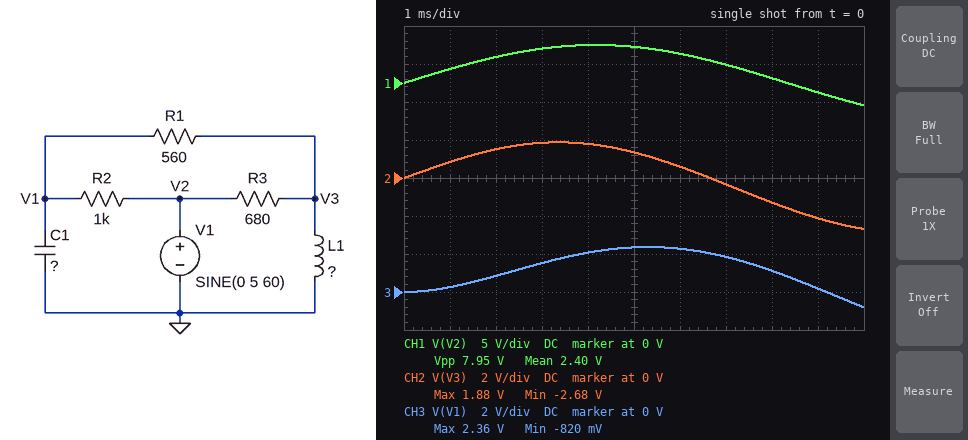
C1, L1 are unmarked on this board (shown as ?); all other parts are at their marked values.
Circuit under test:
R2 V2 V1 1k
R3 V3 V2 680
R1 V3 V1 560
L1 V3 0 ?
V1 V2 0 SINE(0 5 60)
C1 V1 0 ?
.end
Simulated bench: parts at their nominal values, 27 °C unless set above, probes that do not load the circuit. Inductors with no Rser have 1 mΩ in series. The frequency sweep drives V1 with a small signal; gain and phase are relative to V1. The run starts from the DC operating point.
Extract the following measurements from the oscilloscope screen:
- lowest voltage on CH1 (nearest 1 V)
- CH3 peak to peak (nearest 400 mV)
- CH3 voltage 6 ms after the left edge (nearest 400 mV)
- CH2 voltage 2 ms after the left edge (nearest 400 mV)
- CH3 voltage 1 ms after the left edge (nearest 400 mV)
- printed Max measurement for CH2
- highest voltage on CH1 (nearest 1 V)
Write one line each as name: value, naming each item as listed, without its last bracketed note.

lowest voltage on CH1: -3 V
CH3 peak to peak: 3.2 V
CH3 voltage 6 ms after the left edge: 2.4 V
CH2 voltage 2 ms after the left edge: 1.6 V
CH3 voltage 1 ms after the left edge: 400 mV
printed Max measurement for CH2: 1.88 V
highest voltage on CH1: 5 V
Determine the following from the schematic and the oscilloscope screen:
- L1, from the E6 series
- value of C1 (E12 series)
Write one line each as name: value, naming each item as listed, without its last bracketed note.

L1, from the E6 series: 1 H
value of C1: 5.6 µF
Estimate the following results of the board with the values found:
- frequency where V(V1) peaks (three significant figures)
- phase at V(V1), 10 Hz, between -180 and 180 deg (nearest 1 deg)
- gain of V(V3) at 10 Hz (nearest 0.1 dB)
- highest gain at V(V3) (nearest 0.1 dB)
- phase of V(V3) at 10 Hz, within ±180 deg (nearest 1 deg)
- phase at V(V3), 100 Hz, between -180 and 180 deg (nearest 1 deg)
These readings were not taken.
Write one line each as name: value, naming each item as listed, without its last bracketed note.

frequency where V(V1) peaks: 54.6 Hz
phase at V(V1), 10 Hz, between -180 and 180 deg: 5 deg
gain of V(V3) at 10 Hz: -17.6 dB
highest gain at V(V3): -4.5 dB
phase of V(V3) at 10 Hz, within ±180 deg: 80 deg
phase at V(V3), 100 Hz, between -180 and 180 deg: 10 deg
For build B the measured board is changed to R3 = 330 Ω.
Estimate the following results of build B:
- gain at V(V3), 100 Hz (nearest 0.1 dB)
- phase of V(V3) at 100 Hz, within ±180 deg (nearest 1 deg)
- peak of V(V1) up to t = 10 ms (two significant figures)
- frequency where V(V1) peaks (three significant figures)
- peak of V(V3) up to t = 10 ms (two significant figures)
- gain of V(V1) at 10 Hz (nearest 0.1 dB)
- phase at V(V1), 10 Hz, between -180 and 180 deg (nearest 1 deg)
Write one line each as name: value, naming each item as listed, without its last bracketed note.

gain at V(V3), 100 Hz: -2.7 dB
phase of V(V3) at 100 Hz, within ±180 deg: 8 deg
peak of V(V1) up to t = 10 ms: 2.8 V
frequency where V(V1) peaks: 47.1 Hz
peak of V(V3) up to t = 10 ms: 2.6 V
gain of V(V1) at 10 Hz: -7.6 dB
phase at V(V1), 10 Hz, between -180 and 180 deg: 12 deg
